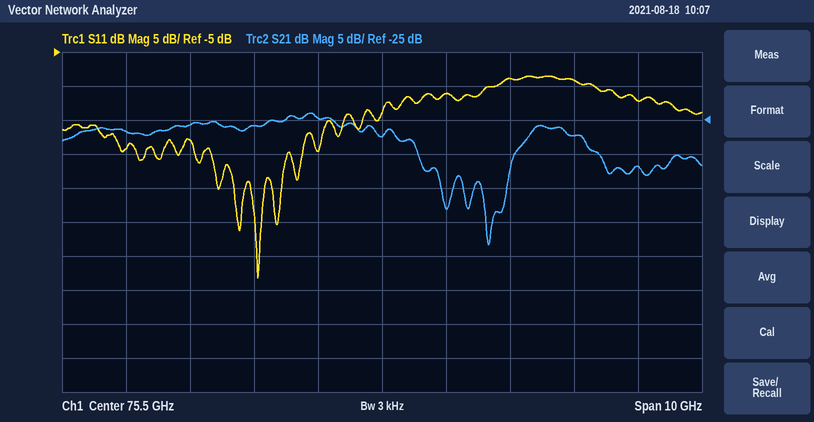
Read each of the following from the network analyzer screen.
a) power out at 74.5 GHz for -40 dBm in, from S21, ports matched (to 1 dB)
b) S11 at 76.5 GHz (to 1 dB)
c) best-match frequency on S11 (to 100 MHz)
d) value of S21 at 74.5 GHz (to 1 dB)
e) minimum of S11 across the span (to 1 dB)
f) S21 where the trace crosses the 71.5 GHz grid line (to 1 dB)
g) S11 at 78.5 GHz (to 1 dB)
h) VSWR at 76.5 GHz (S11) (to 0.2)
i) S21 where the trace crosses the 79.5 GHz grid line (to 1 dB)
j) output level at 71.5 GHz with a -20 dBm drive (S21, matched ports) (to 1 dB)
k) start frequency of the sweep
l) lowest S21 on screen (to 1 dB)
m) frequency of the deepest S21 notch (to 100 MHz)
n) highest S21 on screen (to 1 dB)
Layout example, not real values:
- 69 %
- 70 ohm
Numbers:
- -65 dBm
- -11 dB
- 73.6 GHz
- -25 dB
- -38 dB
- -27 dB
- -9 dB
- 1.8
- -32 dB
- -47 dBm
- 70.5 GHz
- -43 dB
- 77.2 GHz
- -24 dB
